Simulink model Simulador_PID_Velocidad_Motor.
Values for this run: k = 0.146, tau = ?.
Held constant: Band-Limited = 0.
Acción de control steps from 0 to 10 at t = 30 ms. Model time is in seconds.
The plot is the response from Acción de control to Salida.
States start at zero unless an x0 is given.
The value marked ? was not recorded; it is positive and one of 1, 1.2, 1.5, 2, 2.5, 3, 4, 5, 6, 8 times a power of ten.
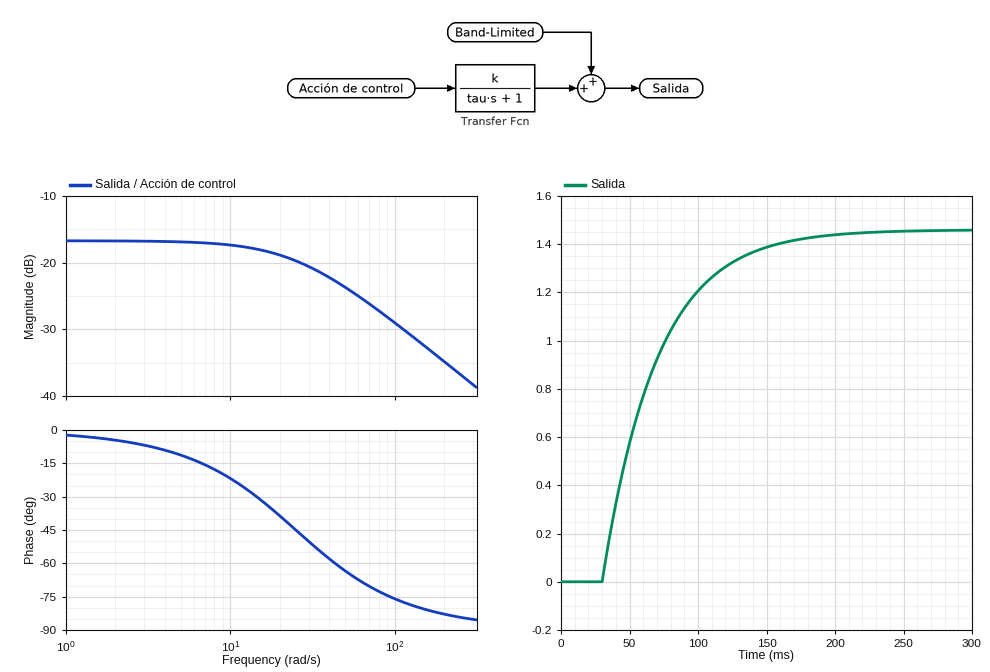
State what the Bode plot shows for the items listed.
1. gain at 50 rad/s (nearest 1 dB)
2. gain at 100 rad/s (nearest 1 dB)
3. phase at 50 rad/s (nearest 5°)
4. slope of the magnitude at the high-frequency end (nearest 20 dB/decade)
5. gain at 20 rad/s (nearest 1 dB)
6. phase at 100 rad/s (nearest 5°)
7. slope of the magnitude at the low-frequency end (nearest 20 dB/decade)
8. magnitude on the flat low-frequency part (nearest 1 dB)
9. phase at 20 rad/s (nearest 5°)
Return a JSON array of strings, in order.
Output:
["-24 dB", "-29 dB", "-65°", "-20 dB/decade", "-19 dB", "-75°", "0 dB/decade", "-17 dB", "-40°"]
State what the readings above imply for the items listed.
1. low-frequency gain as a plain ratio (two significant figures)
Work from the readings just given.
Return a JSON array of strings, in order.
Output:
["0.14"]
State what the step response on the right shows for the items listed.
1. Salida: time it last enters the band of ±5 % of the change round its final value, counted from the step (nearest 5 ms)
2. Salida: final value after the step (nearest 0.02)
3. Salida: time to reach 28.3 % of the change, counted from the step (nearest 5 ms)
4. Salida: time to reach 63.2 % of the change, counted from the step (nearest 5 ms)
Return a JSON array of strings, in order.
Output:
["120 ms", "1.46", "15 ms", "40 ms"]
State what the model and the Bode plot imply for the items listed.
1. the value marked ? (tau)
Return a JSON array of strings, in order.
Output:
["0.04"]
